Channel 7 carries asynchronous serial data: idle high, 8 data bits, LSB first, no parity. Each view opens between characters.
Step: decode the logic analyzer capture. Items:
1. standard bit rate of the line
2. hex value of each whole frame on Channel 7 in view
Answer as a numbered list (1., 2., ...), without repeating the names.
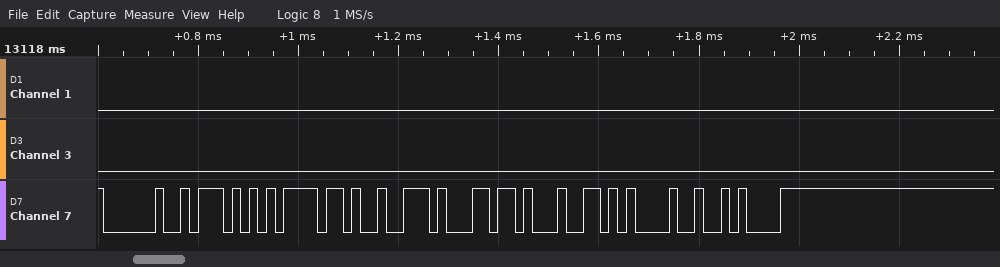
1. 57600 baud
2. 20, 57, 6F, 72, 6C, 64, 21, 0A
